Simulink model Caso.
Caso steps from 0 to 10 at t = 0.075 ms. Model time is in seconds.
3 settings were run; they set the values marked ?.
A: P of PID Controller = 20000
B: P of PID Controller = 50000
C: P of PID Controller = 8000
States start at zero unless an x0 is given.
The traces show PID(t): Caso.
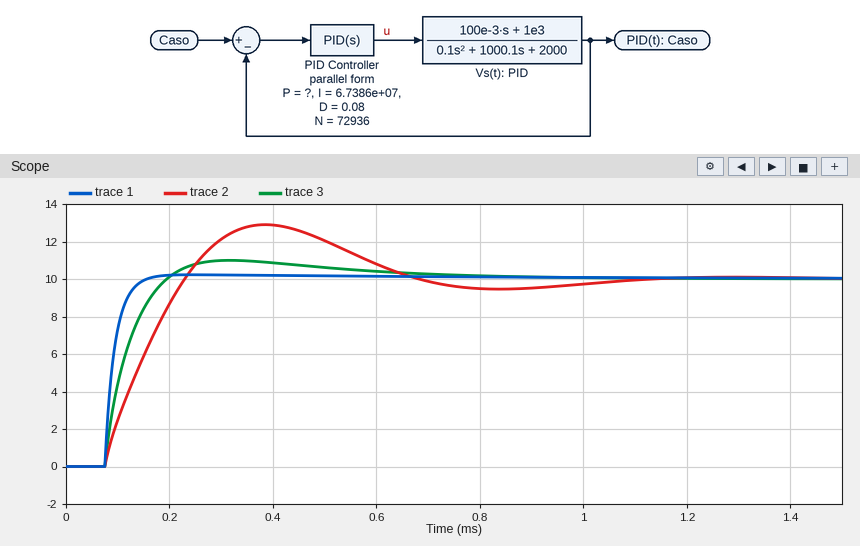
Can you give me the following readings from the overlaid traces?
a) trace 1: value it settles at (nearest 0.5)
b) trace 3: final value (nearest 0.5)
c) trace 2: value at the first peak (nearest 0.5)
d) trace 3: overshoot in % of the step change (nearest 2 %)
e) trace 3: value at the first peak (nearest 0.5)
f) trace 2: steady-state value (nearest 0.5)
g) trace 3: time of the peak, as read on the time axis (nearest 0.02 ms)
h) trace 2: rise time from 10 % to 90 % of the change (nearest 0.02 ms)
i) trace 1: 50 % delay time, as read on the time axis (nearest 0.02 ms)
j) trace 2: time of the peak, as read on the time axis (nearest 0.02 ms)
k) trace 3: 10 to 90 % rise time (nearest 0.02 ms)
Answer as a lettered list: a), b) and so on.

a) 10.0
b) 10.0
c) 13.0
d) 10 %
e) 11.0
f) 10.0
g) 0.32 ms
h) 0.12 ms
i) 0.08 ms
j) 0.38 ms
k) 0.08 ms
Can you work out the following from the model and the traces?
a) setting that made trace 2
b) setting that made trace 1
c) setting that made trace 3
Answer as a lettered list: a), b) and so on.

a) C
b) B
c) A
